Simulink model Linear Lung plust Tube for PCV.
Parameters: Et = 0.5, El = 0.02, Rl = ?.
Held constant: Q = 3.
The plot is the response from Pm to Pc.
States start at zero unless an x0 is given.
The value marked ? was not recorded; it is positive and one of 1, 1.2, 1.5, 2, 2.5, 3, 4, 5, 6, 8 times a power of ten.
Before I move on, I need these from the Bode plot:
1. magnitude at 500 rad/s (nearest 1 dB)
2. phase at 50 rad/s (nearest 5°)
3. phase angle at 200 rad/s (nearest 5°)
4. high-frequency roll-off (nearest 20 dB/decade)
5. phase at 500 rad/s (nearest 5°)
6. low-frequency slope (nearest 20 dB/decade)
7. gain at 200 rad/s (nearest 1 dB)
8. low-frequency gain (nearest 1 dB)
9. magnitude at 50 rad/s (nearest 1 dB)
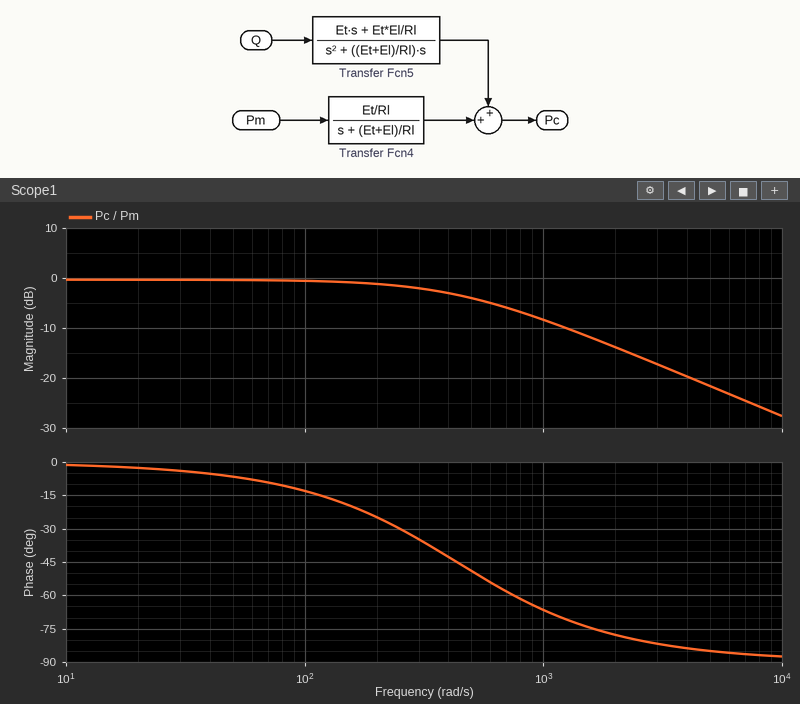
-4 dB
-5°
-25°
-20 dB/decade
-50°
0 dB/decade
-1 dB
0 dB
0 dB
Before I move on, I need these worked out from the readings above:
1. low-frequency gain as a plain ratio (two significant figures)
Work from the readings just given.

1.0
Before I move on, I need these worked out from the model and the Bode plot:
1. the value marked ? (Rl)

0.0012
